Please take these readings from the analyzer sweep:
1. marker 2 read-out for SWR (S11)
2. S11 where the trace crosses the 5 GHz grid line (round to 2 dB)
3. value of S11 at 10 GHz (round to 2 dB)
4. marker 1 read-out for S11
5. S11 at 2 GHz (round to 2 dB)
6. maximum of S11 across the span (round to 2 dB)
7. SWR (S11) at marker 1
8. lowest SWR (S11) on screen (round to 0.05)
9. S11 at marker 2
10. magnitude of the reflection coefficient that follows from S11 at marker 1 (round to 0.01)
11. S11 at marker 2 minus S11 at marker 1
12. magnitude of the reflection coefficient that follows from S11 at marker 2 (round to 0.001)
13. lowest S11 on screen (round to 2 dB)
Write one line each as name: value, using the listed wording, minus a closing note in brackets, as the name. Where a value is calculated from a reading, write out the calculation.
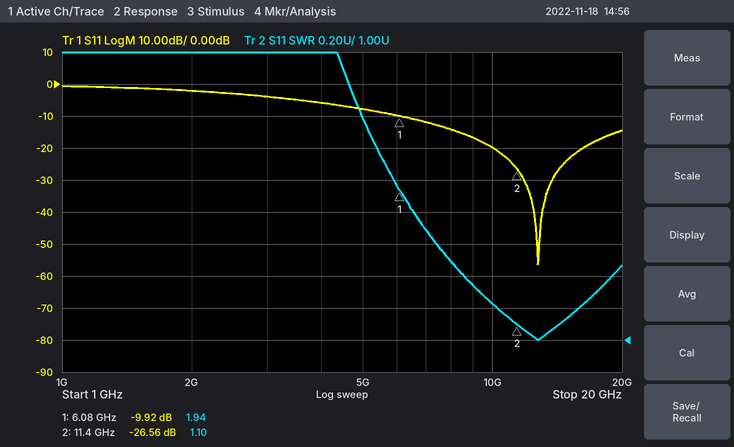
marker 2 read-out for SWR: 1.10
S11 where the trace crosses the 5 GHz grid line: -8 dB
value of S11 at 10 GHz: -20 dB
marker 1 read-out for S11: -9.92 dB
S11 at 2 GHz: -2 dB
maximum of S11 across the span: 0 dB
SWR (S11) at marker 1: 1.94
lowest SWR (S11) on screen: 1.00
S11 at marker 2: -26.56 dB
magnitude of the reflection coefficient that follows from S11 at marker 1: 10^(-9.92/20) ≈ 0.32
S11 at marker 2 minus S11 at marker 1: -26.56 − (-9.92) = -16.64 dB
magnitude of the reflection coefficient that follows from S11 at marker 2: 10^(-26.56/20) ≈ 0.047
lowest S11 on screen: -56 dB
